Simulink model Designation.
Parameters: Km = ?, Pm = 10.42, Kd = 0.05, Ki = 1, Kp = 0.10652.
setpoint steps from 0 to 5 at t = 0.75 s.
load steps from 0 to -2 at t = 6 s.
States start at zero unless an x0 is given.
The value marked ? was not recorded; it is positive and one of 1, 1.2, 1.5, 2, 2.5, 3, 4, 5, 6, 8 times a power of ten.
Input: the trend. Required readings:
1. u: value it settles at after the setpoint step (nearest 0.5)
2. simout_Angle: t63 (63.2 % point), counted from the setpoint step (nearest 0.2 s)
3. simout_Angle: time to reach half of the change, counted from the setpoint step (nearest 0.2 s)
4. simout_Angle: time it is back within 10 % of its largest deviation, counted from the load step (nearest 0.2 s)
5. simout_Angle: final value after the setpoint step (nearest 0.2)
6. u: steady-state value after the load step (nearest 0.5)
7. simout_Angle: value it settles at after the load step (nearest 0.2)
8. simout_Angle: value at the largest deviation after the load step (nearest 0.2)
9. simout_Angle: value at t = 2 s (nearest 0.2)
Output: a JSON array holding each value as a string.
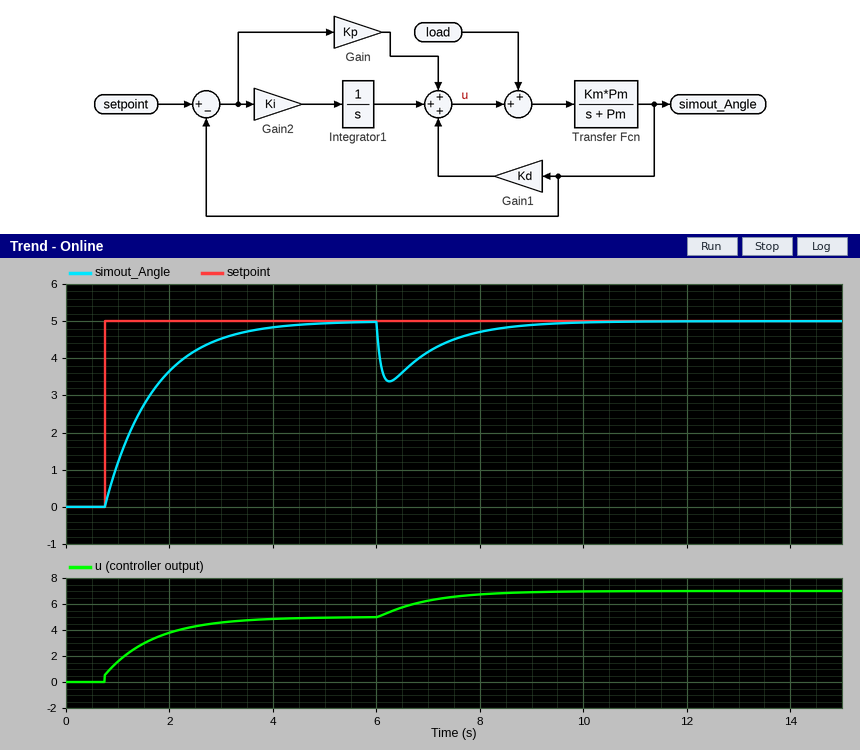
["5.0", "1.0 s", "0.6 s", "2.6 s", "5.0", "7.0", "5.0", "3.4", "3.6"]
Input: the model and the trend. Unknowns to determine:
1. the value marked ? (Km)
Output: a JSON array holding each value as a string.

["1"]
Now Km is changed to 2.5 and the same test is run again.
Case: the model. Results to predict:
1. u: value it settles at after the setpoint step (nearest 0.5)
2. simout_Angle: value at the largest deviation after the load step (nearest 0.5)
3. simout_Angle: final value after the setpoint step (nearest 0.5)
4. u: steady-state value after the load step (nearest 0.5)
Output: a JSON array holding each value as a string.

["2.0", "1.5", "5.0", "4.0"]
